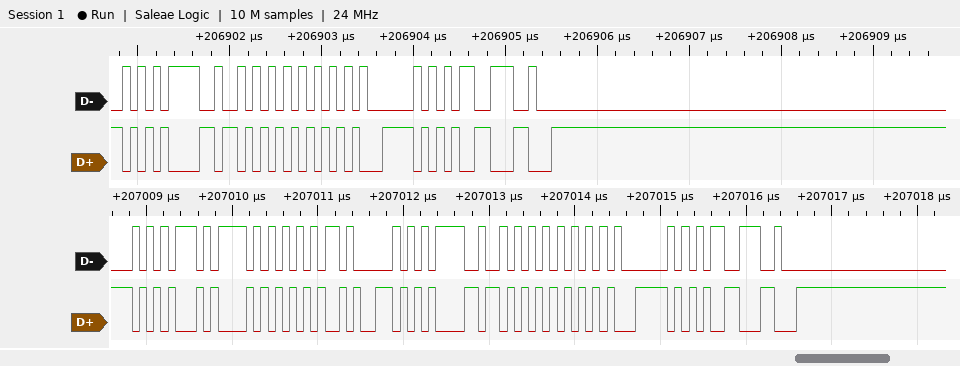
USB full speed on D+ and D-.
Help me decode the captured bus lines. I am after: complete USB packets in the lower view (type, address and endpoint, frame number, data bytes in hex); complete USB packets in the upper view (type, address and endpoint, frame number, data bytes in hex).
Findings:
OUT ADDR 0 EP 0, DATA1 [ ], NAK
DATA1 [ ], NAK
